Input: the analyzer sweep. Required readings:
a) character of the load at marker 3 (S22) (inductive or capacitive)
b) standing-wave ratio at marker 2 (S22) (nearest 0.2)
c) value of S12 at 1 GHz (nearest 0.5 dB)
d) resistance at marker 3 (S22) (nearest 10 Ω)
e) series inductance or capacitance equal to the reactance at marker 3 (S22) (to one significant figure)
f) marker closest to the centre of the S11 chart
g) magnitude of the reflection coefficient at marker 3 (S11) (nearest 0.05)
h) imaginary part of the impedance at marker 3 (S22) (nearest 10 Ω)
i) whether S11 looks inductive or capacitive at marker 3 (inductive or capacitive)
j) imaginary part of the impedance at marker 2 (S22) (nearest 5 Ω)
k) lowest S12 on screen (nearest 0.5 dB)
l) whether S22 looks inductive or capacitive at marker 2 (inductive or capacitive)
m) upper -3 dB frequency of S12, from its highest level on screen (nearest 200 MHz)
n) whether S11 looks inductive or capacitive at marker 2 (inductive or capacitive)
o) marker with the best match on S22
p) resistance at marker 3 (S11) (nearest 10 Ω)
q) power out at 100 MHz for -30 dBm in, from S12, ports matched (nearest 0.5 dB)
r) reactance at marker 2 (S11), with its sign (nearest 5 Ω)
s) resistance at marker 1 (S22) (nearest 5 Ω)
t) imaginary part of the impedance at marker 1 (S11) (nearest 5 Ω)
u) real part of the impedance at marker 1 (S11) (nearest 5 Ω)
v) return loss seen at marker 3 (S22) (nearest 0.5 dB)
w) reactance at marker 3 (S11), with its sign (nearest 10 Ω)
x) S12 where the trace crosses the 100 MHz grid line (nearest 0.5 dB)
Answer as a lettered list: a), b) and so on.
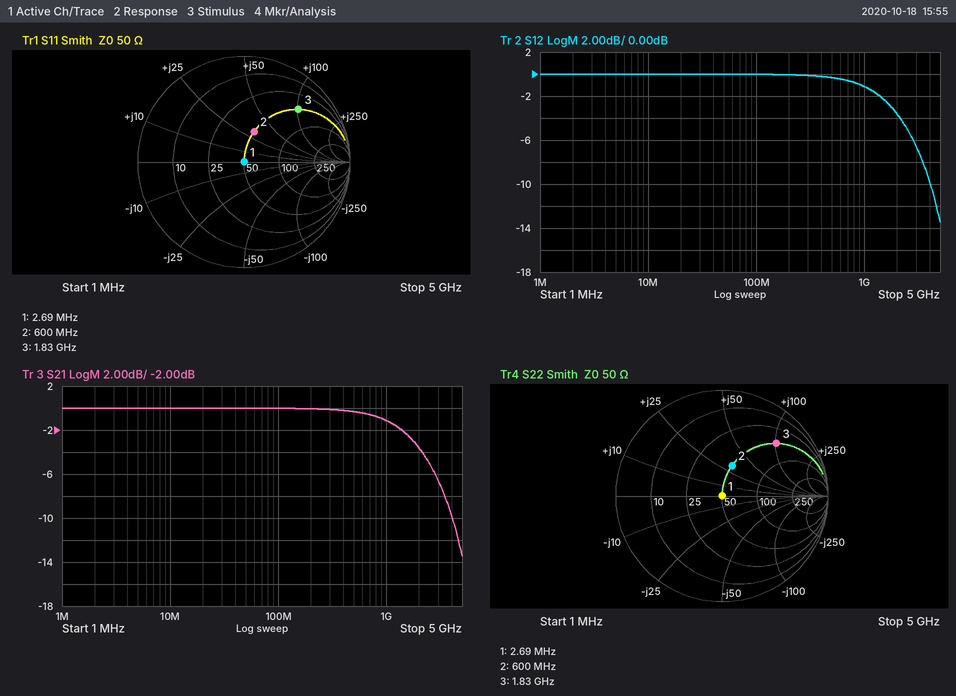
a) inductive
b) 1.8
c) -1.0 dB
d) 50 Ω
e) 9 nH
f) marker 1
g) 0.70
h) +100 Ω
i) inductive
j) +30 Ω
k) -13.5 dB
l) inductive
m) 1.8 GHz
n) inductive
o) marker 1
p) 50 Ω
q) -30.0 dBm
r) +30 Ω
s) 50 Ω
t) 0 Ω
u) 50 Ω
v) 3.0 dB
w) +100 Ω
x) 0.0 dB
